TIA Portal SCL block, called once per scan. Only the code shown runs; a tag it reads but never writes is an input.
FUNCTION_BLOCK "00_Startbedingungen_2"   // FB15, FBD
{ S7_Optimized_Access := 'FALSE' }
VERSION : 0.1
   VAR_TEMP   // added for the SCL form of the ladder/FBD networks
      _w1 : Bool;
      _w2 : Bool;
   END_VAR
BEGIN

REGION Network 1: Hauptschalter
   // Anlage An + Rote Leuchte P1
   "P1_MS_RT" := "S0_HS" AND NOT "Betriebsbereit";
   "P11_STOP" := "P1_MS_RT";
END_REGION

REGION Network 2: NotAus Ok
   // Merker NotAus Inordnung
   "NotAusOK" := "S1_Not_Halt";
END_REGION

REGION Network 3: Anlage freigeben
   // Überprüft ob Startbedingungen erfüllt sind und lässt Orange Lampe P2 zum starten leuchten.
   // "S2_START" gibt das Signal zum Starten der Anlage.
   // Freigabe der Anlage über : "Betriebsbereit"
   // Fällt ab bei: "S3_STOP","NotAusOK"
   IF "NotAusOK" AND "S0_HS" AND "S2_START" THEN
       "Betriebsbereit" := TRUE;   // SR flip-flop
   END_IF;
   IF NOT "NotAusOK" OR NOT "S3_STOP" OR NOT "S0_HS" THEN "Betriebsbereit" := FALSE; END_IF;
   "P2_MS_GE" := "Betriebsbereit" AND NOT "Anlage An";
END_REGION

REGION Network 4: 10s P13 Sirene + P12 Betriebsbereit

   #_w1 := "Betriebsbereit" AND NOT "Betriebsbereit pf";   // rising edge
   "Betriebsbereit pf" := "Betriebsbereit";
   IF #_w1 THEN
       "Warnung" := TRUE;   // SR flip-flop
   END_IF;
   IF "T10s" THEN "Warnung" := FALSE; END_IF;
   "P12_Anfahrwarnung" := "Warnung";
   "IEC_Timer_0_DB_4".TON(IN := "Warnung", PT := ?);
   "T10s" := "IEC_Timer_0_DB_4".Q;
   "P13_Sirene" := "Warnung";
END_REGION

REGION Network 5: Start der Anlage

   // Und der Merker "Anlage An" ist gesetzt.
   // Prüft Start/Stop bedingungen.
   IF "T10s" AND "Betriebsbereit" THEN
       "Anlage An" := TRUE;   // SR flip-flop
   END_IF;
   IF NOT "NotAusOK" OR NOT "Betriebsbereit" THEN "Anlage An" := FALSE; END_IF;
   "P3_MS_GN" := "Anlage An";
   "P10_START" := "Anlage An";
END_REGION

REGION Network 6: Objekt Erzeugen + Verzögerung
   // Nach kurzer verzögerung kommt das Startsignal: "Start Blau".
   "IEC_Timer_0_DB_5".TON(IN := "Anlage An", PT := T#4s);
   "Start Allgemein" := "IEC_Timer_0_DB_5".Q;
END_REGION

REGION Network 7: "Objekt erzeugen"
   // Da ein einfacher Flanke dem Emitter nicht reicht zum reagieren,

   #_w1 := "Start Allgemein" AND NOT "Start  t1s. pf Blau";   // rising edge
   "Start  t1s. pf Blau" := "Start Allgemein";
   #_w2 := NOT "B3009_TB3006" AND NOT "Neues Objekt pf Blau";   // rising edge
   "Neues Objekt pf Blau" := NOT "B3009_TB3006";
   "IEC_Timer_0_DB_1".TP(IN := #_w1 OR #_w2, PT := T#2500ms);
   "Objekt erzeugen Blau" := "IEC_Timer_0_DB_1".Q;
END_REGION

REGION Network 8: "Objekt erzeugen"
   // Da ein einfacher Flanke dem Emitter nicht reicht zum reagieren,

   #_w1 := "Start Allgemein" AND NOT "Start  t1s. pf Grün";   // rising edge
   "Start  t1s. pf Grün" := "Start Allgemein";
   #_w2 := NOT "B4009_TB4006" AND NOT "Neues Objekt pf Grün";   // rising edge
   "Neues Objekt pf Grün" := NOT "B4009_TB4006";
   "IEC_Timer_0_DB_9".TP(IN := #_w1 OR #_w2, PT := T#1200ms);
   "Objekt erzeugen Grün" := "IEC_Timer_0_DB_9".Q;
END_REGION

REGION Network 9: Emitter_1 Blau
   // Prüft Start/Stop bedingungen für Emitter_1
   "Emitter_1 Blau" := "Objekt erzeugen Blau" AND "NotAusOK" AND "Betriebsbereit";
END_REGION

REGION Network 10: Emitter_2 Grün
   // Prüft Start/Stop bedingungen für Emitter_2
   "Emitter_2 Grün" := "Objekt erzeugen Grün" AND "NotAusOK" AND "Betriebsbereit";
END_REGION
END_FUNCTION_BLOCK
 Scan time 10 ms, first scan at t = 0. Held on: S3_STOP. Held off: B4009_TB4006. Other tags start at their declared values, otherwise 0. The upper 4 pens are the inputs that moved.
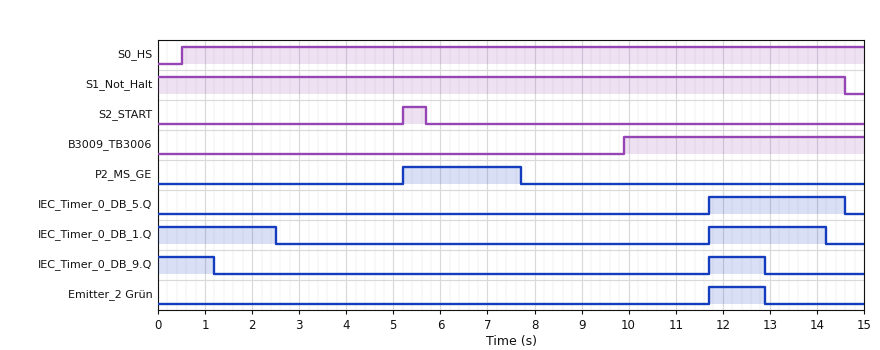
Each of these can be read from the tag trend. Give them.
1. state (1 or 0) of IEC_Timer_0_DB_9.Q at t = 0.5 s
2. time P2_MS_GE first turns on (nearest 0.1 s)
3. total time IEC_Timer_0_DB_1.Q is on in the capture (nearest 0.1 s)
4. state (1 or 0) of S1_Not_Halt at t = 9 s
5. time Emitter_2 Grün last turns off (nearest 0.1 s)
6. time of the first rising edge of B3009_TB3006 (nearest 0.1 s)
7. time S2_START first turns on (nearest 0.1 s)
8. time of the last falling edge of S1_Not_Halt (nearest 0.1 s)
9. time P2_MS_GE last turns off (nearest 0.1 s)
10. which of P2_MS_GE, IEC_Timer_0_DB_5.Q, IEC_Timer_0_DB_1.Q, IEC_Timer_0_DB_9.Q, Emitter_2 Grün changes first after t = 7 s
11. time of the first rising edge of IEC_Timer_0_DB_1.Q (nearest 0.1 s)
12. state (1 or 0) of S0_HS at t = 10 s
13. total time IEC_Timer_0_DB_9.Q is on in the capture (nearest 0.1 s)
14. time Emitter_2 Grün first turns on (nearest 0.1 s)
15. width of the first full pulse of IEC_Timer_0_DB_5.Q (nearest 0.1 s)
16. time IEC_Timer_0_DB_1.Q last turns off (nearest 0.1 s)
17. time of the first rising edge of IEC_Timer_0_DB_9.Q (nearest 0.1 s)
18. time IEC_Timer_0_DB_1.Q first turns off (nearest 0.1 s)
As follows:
1
5.2 s
5.0 s
1
12.9 s
9.9 s
5.2 s
14.6 s
7.7 s
P2_MS_GE
11.7 s
1
2.4 s
11.7 s
2.9 s
14.2 s
11.7 s
2.5 s
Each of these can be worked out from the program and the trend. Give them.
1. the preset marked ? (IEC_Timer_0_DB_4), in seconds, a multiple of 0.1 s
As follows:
2.5 s
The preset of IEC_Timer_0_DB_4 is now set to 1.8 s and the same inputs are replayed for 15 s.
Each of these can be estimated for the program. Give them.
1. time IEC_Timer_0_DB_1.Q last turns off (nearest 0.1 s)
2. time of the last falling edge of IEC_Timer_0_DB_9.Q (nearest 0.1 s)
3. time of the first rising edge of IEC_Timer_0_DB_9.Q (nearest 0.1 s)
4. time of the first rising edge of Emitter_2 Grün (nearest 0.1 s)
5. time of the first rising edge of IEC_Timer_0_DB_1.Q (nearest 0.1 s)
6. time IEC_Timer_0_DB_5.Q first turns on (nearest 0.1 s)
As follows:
13.5 s
12.2 s
11.0 s
11.0 s
11.0 s
11.0 s
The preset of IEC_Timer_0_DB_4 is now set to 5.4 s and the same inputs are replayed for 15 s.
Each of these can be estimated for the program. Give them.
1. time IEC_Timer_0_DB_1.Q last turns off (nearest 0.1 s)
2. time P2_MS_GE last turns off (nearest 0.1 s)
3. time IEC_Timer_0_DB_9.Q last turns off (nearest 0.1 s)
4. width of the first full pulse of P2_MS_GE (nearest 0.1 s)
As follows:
2.5 s
10.6 s
1.2 s
5.4 s
